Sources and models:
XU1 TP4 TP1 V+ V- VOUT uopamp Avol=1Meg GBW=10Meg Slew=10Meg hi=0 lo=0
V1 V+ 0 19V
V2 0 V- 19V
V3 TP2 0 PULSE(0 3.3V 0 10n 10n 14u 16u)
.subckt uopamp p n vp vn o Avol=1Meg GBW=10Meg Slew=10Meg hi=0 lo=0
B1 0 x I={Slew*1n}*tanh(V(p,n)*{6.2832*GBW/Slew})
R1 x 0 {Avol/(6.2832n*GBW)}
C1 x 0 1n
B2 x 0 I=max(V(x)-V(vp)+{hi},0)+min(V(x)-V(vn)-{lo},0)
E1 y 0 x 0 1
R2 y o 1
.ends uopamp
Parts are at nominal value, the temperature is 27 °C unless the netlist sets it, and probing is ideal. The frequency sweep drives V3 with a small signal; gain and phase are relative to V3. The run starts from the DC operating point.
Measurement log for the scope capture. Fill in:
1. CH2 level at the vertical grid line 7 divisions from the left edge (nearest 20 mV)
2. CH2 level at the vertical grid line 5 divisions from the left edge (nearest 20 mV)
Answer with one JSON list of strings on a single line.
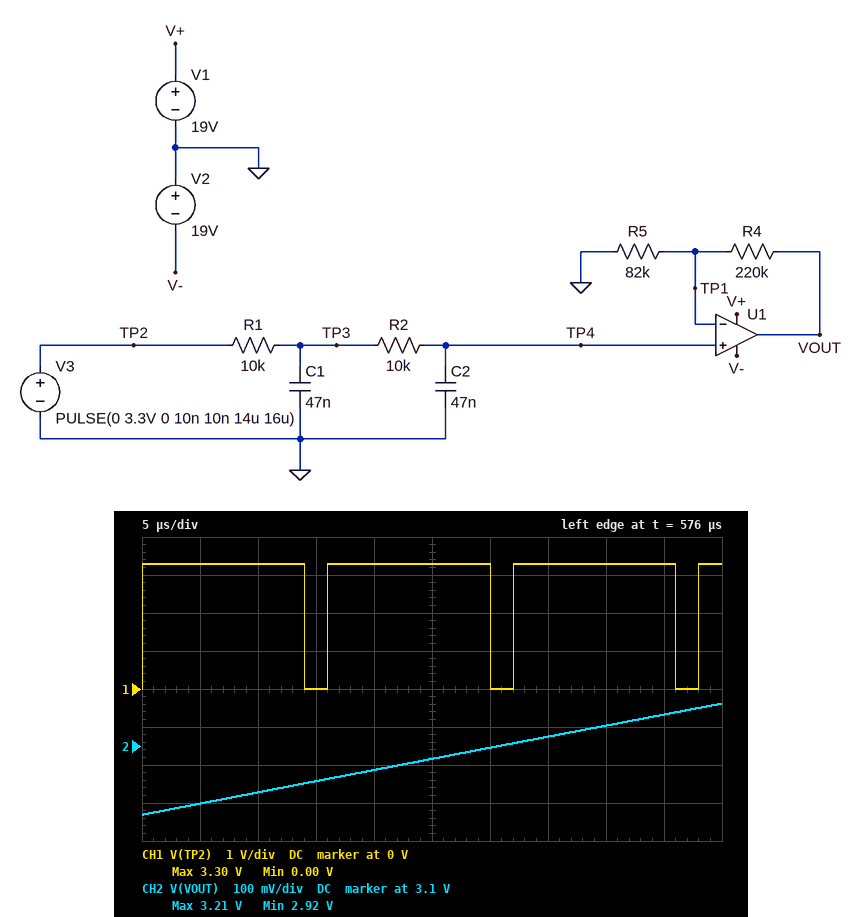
["3.12 V", "3.06 V"]
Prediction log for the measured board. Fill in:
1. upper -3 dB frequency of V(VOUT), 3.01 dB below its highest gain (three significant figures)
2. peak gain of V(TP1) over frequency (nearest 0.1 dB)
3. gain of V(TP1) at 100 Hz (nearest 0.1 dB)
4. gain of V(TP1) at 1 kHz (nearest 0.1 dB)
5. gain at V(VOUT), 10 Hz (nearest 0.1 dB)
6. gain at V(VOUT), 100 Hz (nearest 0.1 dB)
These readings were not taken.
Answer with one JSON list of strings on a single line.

["127 Hz", "0 dB", "-2.1 dB", "-21.4 dB", "11.3 dB", "9.2 dB"]
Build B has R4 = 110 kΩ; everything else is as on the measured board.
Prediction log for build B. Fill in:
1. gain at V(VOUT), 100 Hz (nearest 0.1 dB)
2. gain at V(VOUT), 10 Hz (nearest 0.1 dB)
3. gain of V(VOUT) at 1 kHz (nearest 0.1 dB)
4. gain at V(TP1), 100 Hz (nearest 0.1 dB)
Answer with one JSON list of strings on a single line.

["5.3 dB", "7.4 dB", "-14.0 dB", "-2.1 dB"]
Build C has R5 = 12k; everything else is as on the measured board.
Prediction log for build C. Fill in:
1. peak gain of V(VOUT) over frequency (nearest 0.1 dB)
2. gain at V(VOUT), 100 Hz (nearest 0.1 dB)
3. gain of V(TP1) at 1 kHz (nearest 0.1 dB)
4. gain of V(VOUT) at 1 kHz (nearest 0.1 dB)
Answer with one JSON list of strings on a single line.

["25.7 dB", "23.6 dB", "-21.4 dB", "4.3 dB"]
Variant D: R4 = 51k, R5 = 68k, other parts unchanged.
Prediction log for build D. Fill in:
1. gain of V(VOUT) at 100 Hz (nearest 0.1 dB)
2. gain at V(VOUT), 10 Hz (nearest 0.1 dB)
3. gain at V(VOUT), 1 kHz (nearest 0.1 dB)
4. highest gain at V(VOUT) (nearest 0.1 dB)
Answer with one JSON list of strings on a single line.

["2.8 dB", "4.8 dB", "-16.5 dB", "4.9 dB"]
